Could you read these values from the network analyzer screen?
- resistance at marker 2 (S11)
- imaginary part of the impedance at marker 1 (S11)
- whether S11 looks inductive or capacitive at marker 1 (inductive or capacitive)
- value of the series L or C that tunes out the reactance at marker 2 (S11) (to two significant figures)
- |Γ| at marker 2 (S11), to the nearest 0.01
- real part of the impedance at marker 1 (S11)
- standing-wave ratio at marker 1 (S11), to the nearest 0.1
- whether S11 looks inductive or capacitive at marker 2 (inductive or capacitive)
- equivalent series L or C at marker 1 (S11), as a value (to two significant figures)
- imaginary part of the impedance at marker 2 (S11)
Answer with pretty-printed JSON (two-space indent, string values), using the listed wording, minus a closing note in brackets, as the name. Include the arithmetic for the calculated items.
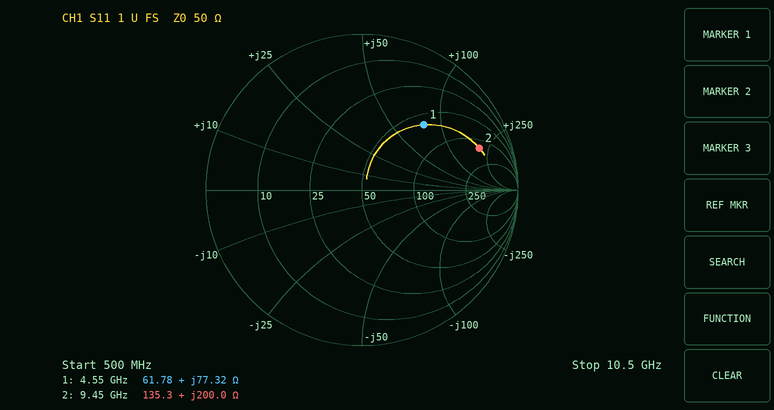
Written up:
{
  "resistance at marker 2": "135.3 Ω",
  "imaginary part of the impedance at marker 1": "+77.32 Ω",
  "whether S11 looks inductive or capacitive at marker 1": "inductive",
  "value of the series L or C that tunes out the reactance at marker 2 (S11)": "C = 1/(2π × 9.45 GHz × 200 Ω) ≈ 84 fF",
  "|Γ| at marker 2 (S11), to the nearest 0.01": "0.80",
  "real part of the impedance at marker 1": "61.78 Ω",
  "standing-wave ratio at marker 1 (S11), to the nearest 0.1": "3.7",
  "whether S11 looks inductive or capacitive at marker 2": "inductive",
  "equivalent series L or C at marker 1 (S11), as a value": "L = 77.32 Ω/(2π × 4.55 GHz) ≈ 2.7 nH",
  "imaginary part of the impedance at marker 2": "+200.0 Ω"
}
